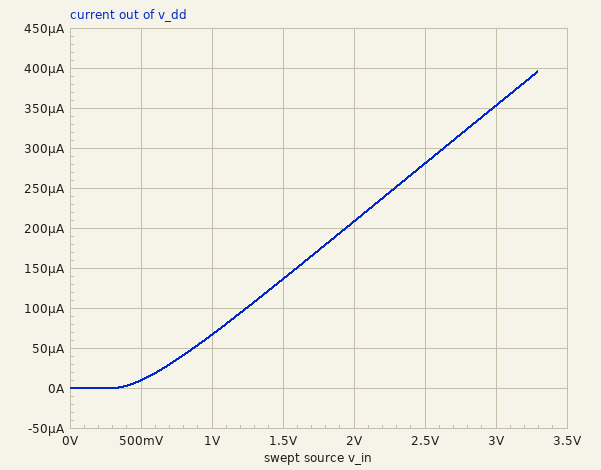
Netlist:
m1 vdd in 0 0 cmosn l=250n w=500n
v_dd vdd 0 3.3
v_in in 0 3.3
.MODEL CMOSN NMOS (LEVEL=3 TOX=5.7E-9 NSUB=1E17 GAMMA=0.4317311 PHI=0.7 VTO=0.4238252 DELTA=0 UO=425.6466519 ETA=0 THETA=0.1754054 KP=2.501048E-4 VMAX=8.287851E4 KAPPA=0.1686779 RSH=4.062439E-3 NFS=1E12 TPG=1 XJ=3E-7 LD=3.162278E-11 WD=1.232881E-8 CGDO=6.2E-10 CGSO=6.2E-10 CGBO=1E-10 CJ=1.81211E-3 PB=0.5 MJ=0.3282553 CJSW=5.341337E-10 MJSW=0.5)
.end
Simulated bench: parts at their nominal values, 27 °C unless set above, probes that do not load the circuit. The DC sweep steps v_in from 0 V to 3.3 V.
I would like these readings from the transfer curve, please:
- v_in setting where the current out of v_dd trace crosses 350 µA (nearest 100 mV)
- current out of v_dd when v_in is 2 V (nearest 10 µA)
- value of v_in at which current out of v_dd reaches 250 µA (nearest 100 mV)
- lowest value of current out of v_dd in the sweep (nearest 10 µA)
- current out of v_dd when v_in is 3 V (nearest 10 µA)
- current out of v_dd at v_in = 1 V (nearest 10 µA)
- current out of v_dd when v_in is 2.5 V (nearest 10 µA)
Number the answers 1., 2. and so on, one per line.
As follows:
1. 3.0 V
2. 210 µA
3. 2.3 V
4. 0 A
5. 350 µA
6. 70 µA
7. 280 µA
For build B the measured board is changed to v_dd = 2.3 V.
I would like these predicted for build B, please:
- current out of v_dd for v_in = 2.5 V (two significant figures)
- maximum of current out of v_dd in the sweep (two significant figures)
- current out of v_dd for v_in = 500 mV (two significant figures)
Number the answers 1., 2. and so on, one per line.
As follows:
1. 260 µA
2. 360 µA
3. 9.0 µA
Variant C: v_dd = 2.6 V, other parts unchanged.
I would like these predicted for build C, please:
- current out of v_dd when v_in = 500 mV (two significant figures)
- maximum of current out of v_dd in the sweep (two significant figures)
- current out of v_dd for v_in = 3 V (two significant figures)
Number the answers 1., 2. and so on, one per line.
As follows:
1. 9.2 µA
2. 370 µA
3. 330 µA
